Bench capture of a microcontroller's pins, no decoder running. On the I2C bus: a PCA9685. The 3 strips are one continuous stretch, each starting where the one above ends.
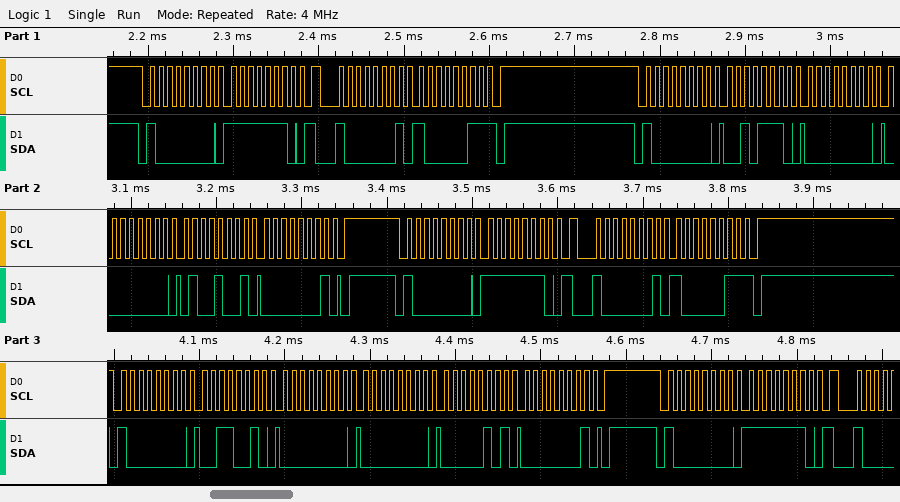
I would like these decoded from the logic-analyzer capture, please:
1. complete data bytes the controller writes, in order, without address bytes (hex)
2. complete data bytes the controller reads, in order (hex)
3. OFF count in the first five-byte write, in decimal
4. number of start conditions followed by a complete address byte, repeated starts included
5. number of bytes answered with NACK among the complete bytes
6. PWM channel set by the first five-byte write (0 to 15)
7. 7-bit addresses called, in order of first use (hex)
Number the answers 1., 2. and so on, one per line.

1. FE 2E 00 00 49 01 FE 32 00 00 05 01 FE
2. 83 83
3. 329
4. 7
5. 2
6. 10
7. 0x40
